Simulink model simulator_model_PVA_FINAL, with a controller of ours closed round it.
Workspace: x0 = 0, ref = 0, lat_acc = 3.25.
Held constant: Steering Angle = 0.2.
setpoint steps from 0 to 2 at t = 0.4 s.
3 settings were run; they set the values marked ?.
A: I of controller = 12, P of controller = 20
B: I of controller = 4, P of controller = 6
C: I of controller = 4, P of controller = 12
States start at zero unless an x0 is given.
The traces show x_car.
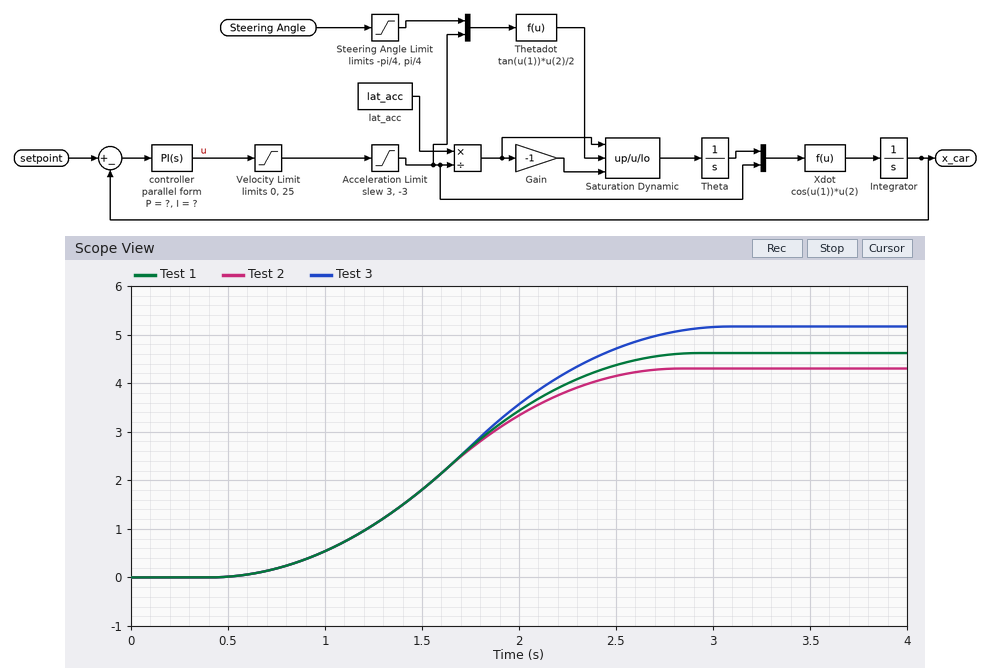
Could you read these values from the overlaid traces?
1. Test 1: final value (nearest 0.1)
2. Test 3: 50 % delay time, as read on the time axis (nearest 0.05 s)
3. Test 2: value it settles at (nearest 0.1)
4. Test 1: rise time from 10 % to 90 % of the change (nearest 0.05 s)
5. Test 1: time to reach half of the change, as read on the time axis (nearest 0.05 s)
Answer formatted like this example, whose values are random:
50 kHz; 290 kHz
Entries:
4.6; 1.70 s; 4.3; 1.40 s; 1.65 s
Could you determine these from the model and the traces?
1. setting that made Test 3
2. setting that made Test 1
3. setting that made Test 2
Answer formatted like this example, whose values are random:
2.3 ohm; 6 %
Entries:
A; B; C
